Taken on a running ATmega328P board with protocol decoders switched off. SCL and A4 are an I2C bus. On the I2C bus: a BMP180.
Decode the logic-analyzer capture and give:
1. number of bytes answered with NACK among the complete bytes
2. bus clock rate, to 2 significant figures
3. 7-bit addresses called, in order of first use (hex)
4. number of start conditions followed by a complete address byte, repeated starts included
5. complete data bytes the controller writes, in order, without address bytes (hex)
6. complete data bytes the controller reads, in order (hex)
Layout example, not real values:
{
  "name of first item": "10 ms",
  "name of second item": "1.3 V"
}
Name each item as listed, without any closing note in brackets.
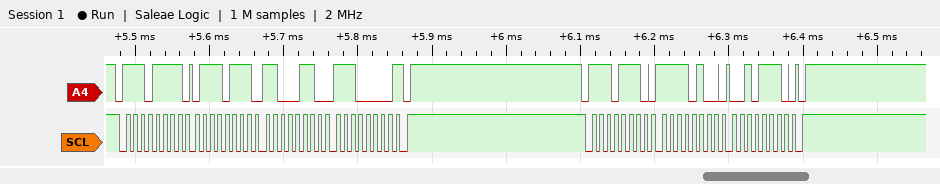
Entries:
{
  "number of bytes answered with NACK among the complete bytes": "1",
  "bus clock rate, to 2 significant figures": "100 kHz",
  "7-bit addresses called, in order of first use": "0x77",
  "number of start conditions followed by a complete address byte, repeated starts included": "2",
  "complete data bytes the controller writes, in order, without address bytes": "F4 2E",
  "complete data bytes the controller reads, in order": "77 C6 E0"
}
